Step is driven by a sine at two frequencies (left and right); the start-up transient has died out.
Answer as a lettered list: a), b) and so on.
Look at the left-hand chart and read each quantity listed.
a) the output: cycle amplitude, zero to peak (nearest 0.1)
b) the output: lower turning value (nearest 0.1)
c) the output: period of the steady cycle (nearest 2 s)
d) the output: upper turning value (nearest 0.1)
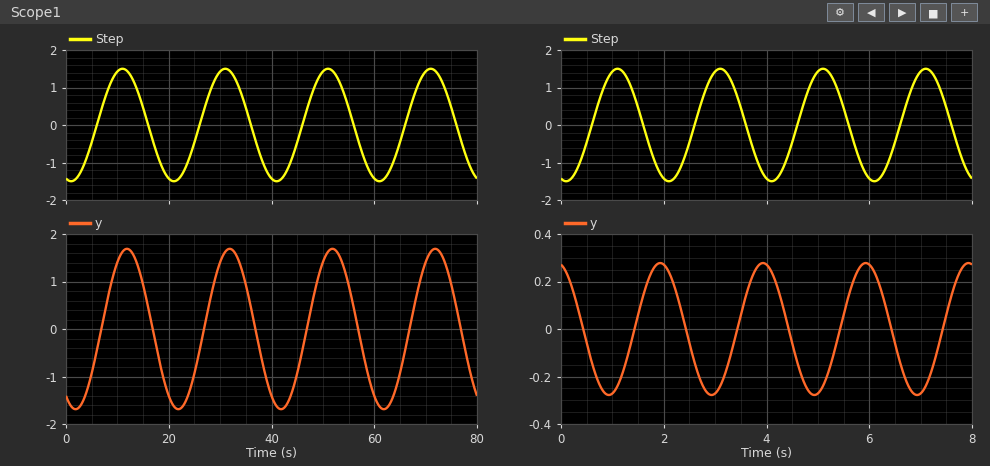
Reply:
a) 1.7
b) -1.7
c) 20 s
d) 1.7
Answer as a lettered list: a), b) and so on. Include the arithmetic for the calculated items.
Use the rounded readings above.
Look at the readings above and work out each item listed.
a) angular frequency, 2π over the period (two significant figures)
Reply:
a) 2π / 20 = 0.31 rad/s
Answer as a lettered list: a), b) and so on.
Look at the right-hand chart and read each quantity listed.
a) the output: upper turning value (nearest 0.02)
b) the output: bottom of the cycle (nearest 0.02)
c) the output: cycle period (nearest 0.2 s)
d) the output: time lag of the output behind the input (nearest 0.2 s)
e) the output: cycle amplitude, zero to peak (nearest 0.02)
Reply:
a) 0.28
b) -0.28
c) 2.0 s
d) 0.8 s
e) 0.28
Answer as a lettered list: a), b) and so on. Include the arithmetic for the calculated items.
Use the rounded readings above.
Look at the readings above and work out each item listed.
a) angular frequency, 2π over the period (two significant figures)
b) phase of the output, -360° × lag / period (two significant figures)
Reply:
a) 2π / 2 = 3.1 rad/s
b) -360 × 0.8 / 2 = -140°
